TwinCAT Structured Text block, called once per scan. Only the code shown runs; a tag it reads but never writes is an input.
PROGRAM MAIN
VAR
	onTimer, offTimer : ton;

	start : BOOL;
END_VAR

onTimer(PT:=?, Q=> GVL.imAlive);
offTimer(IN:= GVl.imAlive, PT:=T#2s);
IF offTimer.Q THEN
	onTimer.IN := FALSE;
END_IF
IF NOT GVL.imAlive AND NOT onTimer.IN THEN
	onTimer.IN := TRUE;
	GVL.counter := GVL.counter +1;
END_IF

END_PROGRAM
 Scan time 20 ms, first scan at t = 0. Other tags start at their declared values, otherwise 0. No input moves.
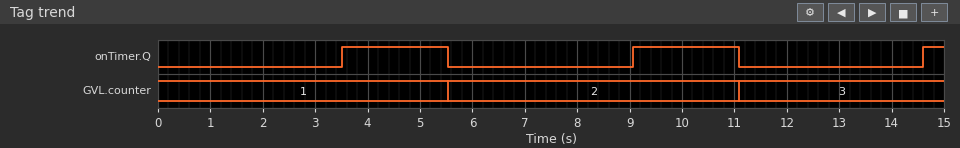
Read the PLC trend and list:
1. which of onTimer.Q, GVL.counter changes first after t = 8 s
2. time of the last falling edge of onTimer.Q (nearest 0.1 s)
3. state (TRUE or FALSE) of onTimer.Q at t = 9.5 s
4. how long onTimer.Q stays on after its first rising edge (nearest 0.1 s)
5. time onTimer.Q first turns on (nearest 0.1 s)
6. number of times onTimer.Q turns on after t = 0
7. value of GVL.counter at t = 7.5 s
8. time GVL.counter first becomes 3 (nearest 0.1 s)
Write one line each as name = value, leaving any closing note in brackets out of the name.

which of onTimer.Q, GVL.counter changes first after t = 8 s = onTimer.Q
time of the last falling edge of onTimer.Q = 11.1 s
state (TRUE or FALSE) of onTimer.Q at t = 9.5 s = TRUE
how long onTimer.Q stays on after its first rising edge = 2.0 s
time onTimer.Q first turns on = 3.5 s
number of times onTimer.Q turns on after t = 0 = 3
value of GVL.counter at t = 7.5 s = 2
time GVL.counter first becomes 3 = 11.1 s
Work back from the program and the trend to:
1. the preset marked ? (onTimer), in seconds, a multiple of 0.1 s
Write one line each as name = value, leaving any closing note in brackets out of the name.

the preset marked ? (onTimer), in seconds, a multiple of 0.1 s = 3.5 s
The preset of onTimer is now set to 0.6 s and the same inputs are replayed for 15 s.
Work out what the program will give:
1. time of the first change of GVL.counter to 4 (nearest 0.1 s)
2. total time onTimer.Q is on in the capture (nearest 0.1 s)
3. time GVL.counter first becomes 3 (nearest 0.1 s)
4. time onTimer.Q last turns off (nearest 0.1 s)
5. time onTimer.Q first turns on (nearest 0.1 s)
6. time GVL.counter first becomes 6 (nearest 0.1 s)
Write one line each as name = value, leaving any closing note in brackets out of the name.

time of the first change of GVL.counter to 4 = 7.9 s
total time onTimer.Q is on in the capture = 11.3 s
time GVL.counter first becomes 3 = 5.3 s
time onTimer.Q last turns off = 13.2 s
time onTimer.Q first turns on = 0.6 s
time GVL.counter first becomes 6 = 13.2 s
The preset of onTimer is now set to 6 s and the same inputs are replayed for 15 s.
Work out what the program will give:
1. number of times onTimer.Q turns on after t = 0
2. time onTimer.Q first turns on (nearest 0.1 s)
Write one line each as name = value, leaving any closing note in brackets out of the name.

number of times onTimer.Q turns on after t = 0 = 2
time onTimer.Q first turns on = 6.0 s
